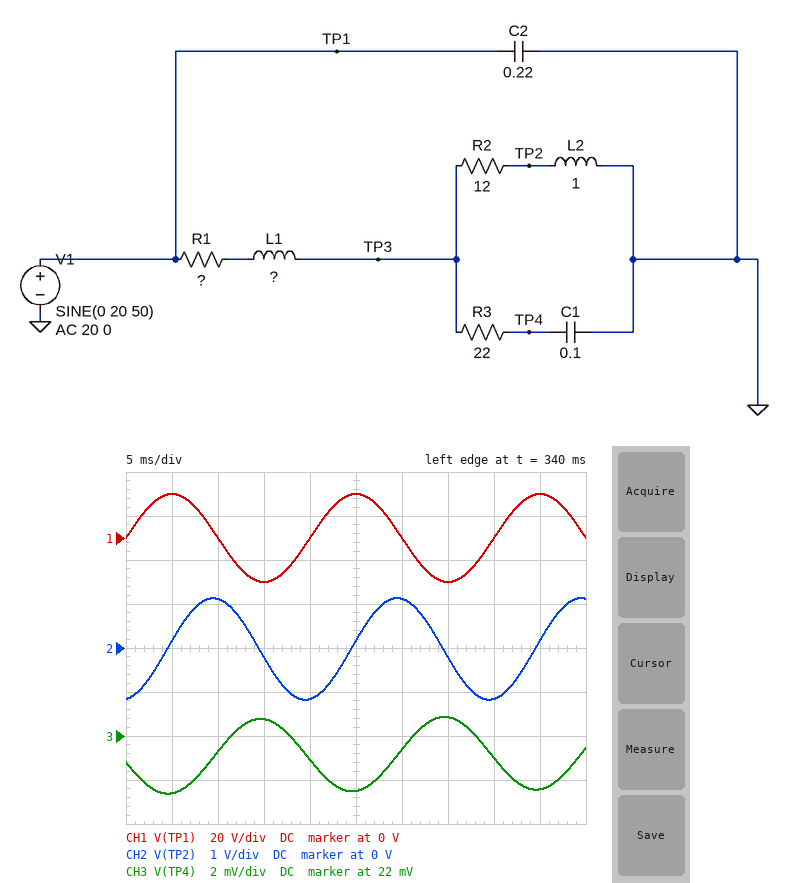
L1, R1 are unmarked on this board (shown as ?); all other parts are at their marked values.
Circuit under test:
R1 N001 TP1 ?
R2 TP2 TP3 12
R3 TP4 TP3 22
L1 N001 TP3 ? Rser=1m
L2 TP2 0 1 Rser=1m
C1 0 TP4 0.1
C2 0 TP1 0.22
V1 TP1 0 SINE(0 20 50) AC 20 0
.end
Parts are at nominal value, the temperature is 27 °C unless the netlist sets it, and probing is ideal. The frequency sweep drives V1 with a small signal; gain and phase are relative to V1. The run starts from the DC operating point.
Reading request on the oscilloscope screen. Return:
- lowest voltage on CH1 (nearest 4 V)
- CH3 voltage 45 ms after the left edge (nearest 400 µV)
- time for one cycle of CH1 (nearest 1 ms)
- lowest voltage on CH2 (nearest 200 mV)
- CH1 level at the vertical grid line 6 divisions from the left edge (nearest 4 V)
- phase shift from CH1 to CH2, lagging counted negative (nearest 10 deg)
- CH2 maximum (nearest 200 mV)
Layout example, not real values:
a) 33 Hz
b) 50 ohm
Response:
a) -20 V
b) 19.6 mV
c) 20 ms
d) -1.2 V
e) 0 V
f) -80 deg
g) 1.2 V
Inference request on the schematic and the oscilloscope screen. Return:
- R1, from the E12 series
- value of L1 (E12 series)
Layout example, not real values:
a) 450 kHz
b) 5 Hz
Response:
a) 0.82 Ω
b) 1.2 H
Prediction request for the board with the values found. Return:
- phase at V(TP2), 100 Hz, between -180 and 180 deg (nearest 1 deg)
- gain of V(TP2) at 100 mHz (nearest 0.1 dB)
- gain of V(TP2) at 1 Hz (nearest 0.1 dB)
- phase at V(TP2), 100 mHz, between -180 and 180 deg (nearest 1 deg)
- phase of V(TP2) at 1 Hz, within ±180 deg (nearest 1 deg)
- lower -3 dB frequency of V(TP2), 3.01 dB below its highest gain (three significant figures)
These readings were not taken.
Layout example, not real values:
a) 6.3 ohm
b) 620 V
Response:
a) -85 deg
b) -26.3 dB
c) -10.5 dB
d) 82 deg
e) 31 deg
f) 667 mHz
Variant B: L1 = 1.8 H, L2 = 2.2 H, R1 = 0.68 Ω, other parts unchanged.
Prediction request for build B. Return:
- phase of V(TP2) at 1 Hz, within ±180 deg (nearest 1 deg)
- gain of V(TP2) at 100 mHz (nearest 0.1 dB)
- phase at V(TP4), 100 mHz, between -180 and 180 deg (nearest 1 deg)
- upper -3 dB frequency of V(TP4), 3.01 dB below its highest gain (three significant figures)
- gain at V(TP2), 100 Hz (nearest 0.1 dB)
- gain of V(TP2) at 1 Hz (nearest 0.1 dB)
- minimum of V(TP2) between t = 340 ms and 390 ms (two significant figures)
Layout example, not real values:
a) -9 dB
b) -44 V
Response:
a) 10 deg
b) -19.4 dB
c) -61 deg
d) 71.5 mHz
e) -34.2 dB
f) -7.2 dB
g) -810 mV
